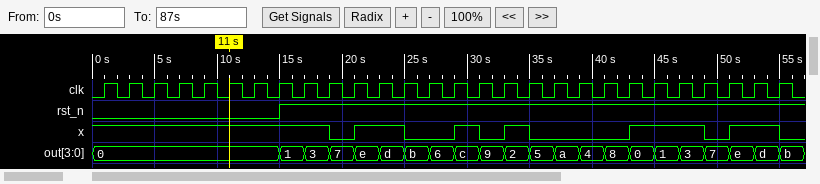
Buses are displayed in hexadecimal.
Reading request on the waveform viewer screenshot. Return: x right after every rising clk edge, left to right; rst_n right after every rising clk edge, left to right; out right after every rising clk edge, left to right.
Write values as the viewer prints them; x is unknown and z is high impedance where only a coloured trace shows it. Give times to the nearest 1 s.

1 1 1 1 1 1 1 1 1 0 1 1 0 0 1 0 1 0 0 0 0 1 1 1 0 1 1 0
0 0 0 0 0 0 0 1 1 1 1 1 1 1 1 1 1 1 1 1 1 1 1 1 1 1 1 1
0, 0, 0, 0, 0, 0, 0, 1, 3, 7, e, d, b, 6, c, 9, 2, 5, a, 4, 8, 0, 1, 3, 7, e, d, b
